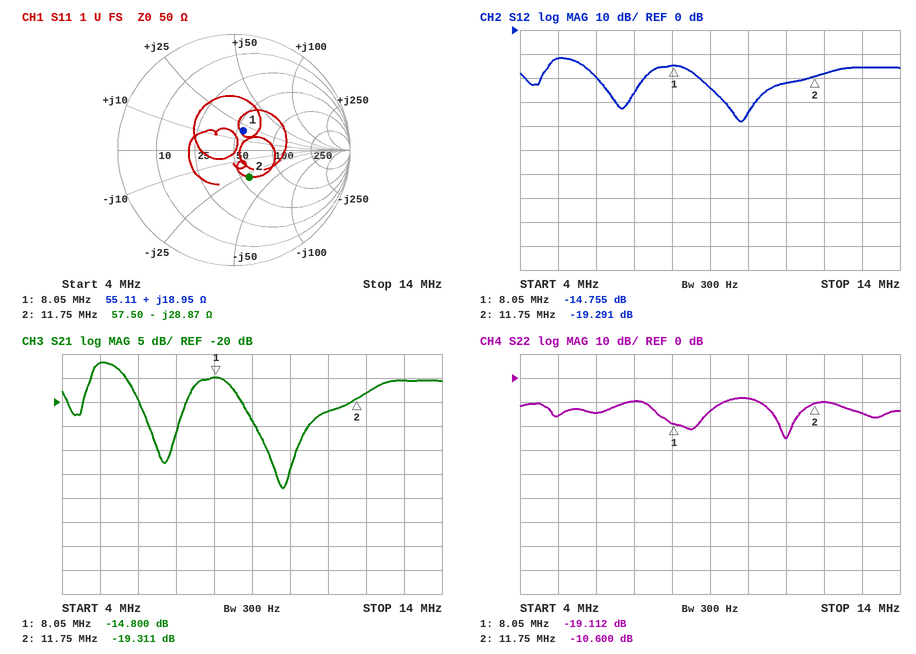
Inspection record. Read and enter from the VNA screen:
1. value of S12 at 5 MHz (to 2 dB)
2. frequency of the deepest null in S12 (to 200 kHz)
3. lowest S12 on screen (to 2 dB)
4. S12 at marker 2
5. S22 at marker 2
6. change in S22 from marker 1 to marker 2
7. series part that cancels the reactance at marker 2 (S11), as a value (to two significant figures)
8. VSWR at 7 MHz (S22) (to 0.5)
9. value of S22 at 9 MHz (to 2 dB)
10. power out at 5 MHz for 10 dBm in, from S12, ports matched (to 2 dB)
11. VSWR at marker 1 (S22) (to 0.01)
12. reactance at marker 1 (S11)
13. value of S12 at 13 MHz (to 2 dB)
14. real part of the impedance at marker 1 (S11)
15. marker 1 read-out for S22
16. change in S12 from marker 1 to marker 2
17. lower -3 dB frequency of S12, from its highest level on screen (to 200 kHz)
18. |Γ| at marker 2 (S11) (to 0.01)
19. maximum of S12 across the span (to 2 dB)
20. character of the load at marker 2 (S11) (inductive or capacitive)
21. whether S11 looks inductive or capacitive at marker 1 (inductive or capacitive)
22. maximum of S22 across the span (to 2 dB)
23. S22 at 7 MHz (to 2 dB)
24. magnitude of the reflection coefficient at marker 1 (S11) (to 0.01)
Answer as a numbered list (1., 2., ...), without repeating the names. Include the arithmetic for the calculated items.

1. -12 dB
2. 9.8 MHz
3. -38 dB
4. -19.291 dB
5. -10.600 dB
6. -10.6 − (-19.112) = 8.512 dB
7. L = 28.87 Ω/(2π × 11.75 MHz) ≈ 391 nH, so 390 nH to two significant figures
8. |Γ| = 10^(-10/20) = 0.3162; VSWR = (1 + 0.3162)/(1 − 0.3162) ≈ 1.92, so 2.0 to the nearest 0.5
9. -14 dB
10. 10 dBm + (-12 dB) = -2 dBm
11. (1 + 0.1108)/(1 − 0.1108) ≈ 1.25
12. +18.95 Ω
13. -16 dB
14. 55.11 Ω
15. -19.112 dB
16. -19.291 − (-14.755) = -4.536 dB
17. 4.8 MHz
18. 0.27
19. -12 dB
20. capacitive
21. inductive
22. -8 dB
23. -10 dB
24. 0.18
